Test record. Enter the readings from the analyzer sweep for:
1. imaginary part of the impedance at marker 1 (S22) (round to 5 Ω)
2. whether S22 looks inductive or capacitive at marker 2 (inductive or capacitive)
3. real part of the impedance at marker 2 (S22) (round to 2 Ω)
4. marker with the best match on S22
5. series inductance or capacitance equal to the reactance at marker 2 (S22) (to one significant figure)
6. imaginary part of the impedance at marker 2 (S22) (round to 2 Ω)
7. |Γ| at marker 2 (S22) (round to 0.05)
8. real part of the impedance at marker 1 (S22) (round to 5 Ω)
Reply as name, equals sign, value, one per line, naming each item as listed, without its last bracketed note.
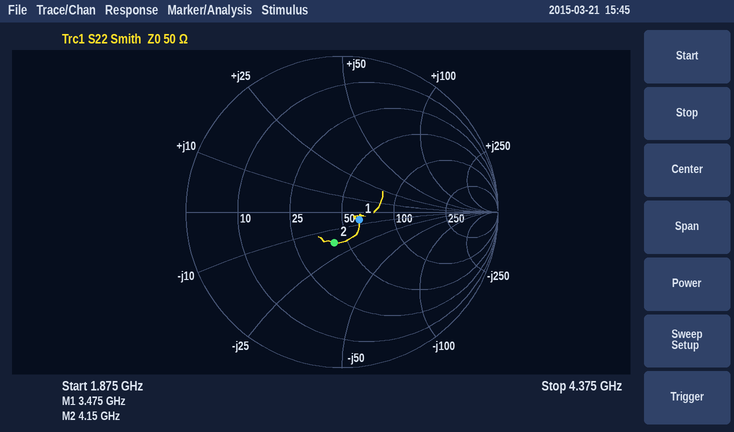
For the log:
imaginary part of the impedance at marker 1 (S22) = -5 Ω
whether S22 looks inductive or capacitive at marker 2 = capacitive
real part of the impedance at marker 2 (S22) = 42 Ω
marker with the best match on S22 = marker 1
series inductance or capacitance equal to the reactance at marker 2 (S22) = 2 pF
imaginary part of the impedance at marker 2 (S22) = -18 Ω
|Γ| at marker 2 (S22) = 0.20
real part of the impedance at marker 1 (S22) = 60 Ω
